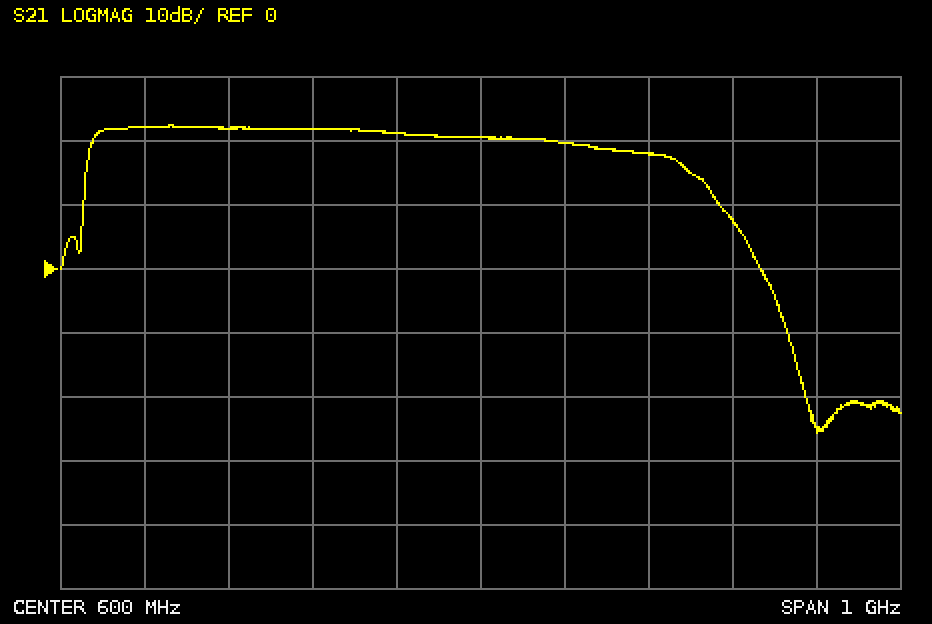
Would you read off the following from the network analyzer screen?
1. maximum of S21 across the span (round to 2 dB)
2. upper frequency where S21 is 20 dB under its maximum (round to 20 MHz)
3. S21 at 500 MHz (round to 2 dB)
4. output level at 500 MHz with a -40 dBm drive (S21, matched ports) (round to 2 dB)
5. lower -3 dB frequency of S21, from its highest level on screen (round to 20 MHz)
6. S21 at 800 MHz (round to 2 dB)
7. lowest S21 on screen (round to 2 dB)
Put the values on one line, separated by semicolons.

22 dB; 920 MHz; 22 dB; -18 dBm; 140 MHz; 18 dB; -26 dB
